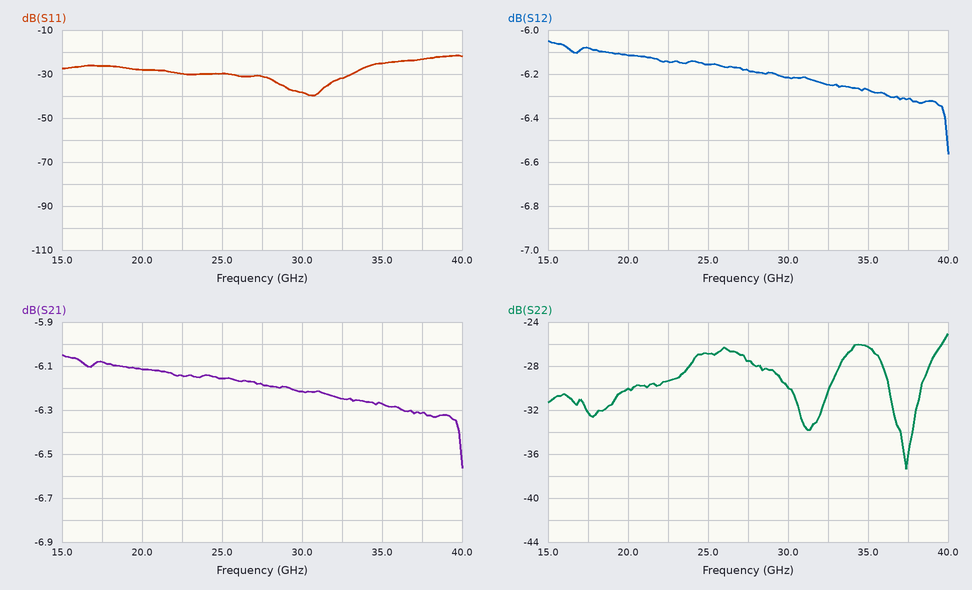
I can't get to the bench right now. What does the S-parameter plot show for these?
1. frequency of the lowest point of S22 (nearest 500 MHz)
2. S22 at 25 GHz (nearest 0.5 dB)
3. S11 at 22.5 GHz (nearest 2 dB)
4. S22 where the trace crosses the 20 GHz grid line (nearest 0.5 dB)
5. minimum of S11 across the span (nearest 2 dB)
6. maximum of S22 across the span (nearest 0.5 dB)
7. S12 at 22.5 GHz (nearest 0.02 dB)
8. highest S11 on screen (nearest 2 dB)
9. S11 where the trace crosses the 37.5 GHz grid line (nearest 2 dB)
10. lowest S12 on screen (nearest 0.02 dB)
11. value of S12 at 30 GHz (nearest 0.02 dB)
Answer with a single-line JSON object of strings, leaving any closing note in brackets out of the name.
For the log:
{"frequency of the lowest point of S22": "37.5 GHz", "S22 at 25 GHz": "-27.0 dB", "S11 at 22.5 GHz": "-30 dB", "S22 where the trace crosses the 20 GHz grid line": "-30.0 dB", "minimum of S11 across the span": "-40 dB", "maximum of S22 across the span": "-25.0 dB", "S12 at 22.5 GHz": "-6.14 dB", "highest S11 on screen": "-22 dB", "S11 where the trace crosses the 37.5 GHz grid line": "-24 dB", "lowest S12 on screen": "-6.56 dB", "value of S12 at 30 GHz": "-6.22 dB"}
